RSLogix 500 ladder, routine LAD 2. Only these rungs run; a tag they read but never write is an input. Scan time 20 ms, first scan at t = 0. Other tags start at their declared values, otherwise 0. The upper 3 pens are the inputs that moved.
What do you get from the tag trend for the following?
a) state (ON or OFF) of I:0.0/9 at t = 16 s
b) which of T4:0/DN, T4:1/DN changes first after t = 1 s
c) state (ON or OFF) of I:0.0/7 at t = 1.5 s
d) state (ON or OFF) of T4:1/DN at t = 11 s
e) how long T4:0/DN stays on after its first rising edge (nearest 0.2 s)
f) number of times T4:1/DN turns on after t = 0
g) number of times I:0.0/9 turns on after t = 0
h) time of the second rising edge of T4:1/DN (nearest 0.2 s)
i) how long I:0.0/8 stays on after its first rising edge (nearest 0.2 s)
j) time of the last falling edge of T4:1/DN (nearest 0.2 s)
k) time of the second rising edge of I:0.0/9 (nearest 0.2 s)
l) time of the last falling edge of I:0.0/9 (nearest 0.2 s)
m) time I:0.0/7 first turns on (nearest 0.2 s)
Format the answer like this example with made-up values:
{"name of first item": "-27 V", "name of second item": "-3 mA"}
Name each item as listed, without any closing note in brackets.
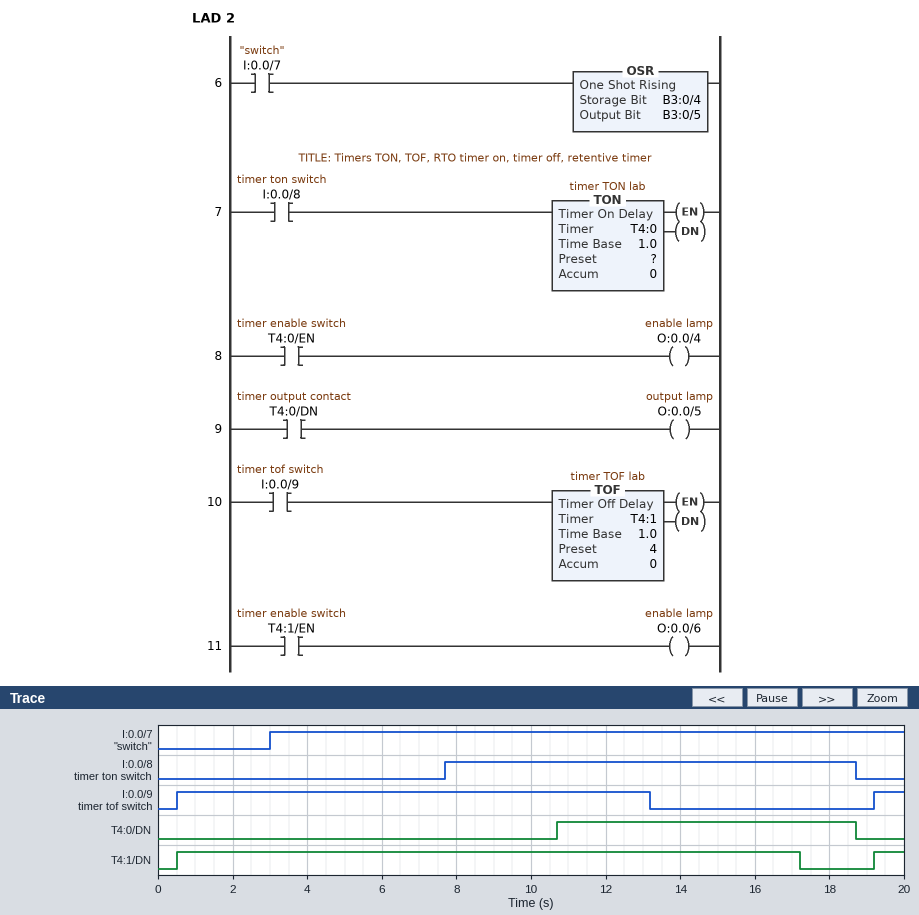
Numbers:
{"state (ON or OFF) of I:0.0/9 at t = 16 s": "OFF", "which of T4:0/DN, T4:1/DN changes first after t = 1 s": "T4:0/DN", "state (ON or OFF) of I:0.0/7 at t = 1.5 s": "OFF", "state (ON or OFF) of T4:1/DN at t = 11 s": "ON", "how long T4:0/DN stays on after its first rising edge": "8.0 s", "number of times T4:1/DN turns on after t = 0": "2", "number of times I:0.0/9 turns on after t = 0": "2", "time of the second rising edge of T4:1/DN": "19.2 s", "how long I:0.0/8 stays on after its first rising edge": "11.0 s", "time of the last falling edge of T4:1/DN": "17.2 s", "time of the second rising edge of I:0.0/9": "19.2 s", "time of the last falling edge of I:0.0/9": "13.2 s", "time I:0.0/7 first turns on": "3.0 s"}
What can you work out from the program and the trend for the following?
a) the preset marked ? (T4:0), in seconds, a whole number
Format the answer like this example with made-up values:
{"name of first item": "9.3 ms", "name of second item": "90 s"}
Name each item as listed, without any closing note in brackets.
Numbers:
{"the preset marked ? (T4:0), in seconds, a whole number": "3 s"}
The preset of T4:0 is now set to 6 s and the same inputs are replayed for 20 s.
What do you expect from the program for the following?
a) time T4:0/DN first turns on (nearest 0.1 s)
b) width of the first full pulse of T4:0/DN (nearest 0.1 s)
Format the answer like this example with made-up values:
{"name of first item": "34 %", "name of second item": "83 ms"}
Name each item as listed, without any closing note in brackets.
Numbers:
{"time T4:0/DN first turns on": "13.7 s", "width of the first full pulse of T4:0/DN": "5.0 s"}
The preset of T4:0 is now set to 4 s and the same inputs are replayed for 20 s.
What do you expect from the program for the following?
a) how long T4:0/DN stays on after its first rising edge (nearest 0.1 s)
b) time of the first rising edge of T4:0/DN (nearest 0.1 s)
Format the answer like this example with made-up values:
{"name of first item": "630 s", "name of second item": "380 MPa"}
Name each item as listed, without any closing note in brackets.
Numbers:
{"how long T4:0/DN stays on after its first rising edge": "7.0 s", "time of the first rising edge of T4:0/DN": "11.7 s"}
